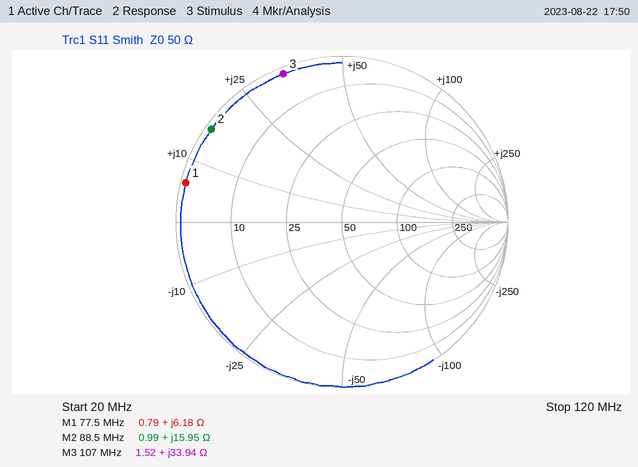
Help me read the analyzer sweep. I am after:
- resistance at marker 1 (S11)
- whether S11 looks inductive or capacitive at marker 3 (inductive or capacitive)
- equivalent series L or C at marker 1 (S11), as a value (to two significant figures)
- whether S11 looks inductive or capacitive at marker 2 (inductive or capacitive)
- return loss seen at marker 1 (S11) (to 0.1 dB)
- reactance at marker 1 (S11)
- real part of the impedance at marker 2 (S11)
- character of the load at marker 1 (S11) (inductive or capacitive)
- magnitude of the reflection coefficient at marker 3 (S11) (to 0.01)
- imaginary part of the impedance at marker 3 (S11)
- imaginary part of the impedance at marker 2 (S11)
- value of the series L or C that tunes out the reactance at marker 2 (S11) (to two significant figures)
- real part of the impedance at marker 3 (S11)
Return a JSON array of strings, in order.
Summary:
["0.79 Ω", "inductive", "13 nH", "inductive", "0.3 dB", "+6.18 Ω", "0.99 Ω", "inductive", "0.96", "+33.94 Ω", "+15.95 Ω", "110 pF", "1.52 Ω"]
